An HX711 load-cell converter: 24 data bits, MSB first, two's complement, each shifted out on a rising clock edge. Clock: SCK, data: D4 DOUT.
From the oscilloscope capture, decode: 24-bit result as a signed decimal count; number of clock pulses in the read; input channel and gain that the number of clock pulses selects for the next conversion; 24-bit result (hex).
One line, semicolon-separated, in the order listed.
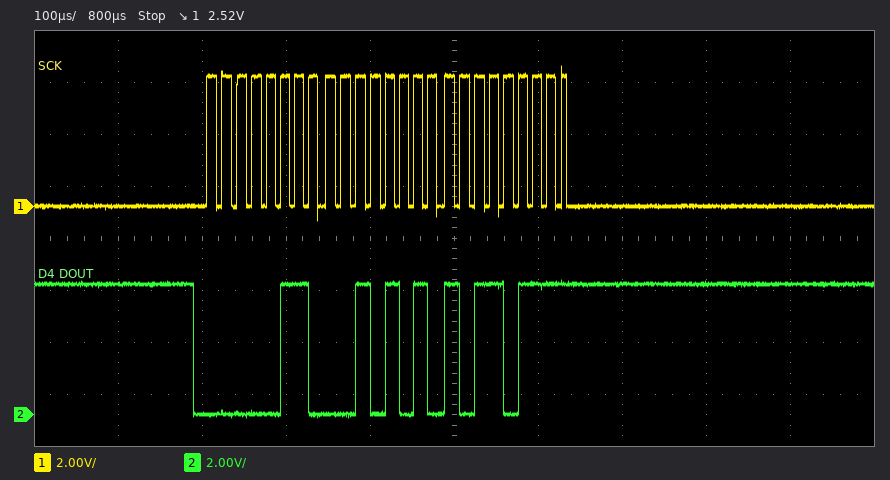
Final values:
404151; 25; channel A, gain 128; 0x062AB7
